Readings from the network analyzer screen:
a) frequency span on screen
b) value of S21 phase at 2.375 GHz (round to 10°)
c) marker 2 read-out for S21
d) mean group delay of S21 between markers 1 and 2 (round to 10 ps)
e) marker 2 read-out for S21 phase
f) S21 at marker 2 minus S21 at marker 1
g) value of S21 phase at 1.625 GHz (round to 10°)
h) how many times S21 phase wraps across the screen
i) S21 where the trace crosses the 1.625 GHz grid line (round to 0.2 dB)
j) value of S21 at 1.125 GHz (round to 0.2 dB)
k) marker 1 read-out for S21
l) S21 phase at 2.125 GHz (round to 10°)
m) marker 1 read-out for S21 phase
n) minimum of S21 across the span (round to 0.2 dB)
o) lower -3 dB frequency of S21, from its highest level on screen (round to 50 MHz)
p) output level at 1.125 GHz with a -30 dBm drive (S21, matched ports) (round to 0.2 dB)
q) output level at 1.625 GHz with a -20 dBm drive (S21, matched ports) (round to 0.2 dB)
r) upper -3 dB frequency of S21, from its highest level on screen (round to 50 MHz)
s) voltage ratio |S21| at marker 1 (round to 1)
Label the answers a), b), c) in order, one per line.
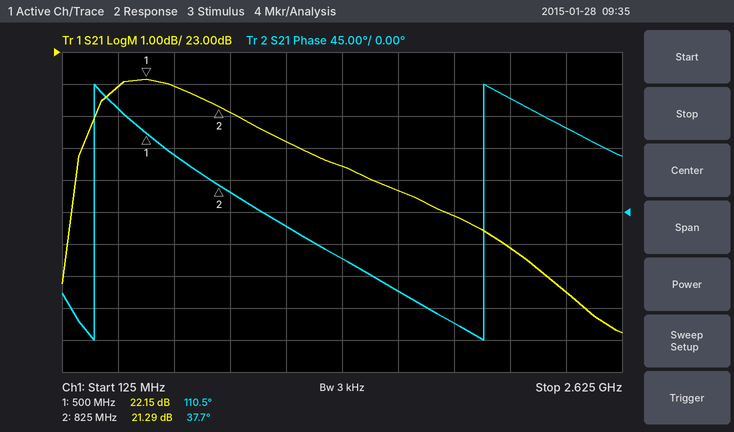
a) 2.5 GHz
b) 120°
c) 21.29 dB
d) 620 ps
e) 37.7°
f) -0.86 dB
g) -110°
h) 2
i) 18.6 dB
j) 20.2 dB
k) 22.15 dB
l) 160°
m) 110.5°
n) 14.2 dB
o) 200 MHz
p) -9.8 dBm
q) -1.4 dBm
r) 1.45 GHz
s) 13
